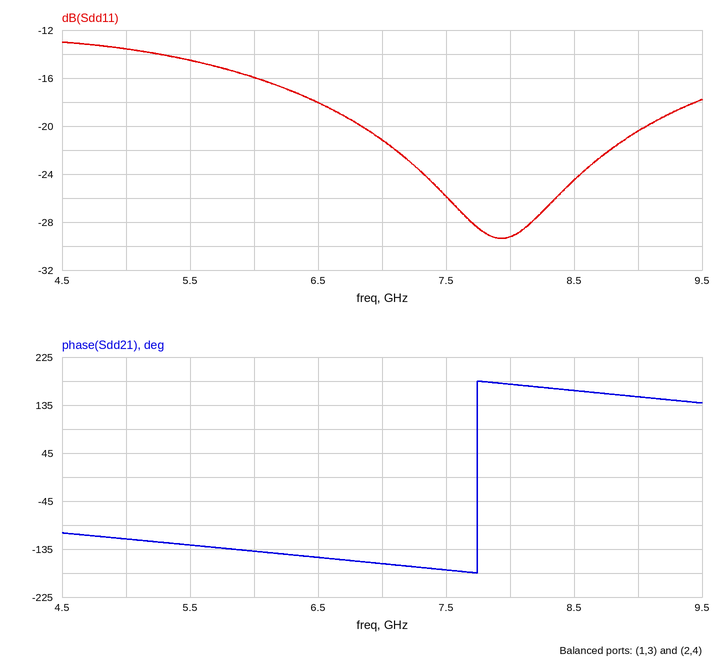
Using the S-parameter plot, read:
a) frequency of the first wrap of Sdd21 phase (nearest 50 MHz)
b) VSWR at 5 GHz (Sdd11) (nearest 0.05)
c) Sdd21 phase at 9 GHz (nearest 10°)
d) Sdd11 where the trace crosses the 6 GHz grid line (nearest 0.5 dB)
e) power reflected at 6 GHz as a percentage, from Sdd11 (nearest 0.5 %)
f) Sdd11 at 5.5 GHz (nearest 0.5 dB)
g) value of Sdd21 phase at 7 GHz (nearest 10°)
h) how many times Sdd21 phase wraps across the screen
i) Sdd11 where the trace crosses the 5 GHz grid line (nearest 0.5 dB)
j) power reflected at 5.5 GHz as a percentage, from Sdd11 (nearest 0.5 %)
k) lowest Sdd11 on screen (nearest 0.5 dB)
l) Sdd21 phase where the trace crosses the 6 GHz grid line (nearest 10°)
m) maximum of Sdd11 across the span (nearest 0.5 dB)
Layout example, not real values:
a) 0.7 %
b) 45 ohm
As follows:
a) 7.75 GHz
b) 1.55
c) 150°
d) -16.0 dB
e) 2.5 %
f) -14.5 dB
g) -160°
h) 1
i) -13.5 dB
j) 3.5 %
k) -29.5 dB
l) -140°
m) -13.0 dB
